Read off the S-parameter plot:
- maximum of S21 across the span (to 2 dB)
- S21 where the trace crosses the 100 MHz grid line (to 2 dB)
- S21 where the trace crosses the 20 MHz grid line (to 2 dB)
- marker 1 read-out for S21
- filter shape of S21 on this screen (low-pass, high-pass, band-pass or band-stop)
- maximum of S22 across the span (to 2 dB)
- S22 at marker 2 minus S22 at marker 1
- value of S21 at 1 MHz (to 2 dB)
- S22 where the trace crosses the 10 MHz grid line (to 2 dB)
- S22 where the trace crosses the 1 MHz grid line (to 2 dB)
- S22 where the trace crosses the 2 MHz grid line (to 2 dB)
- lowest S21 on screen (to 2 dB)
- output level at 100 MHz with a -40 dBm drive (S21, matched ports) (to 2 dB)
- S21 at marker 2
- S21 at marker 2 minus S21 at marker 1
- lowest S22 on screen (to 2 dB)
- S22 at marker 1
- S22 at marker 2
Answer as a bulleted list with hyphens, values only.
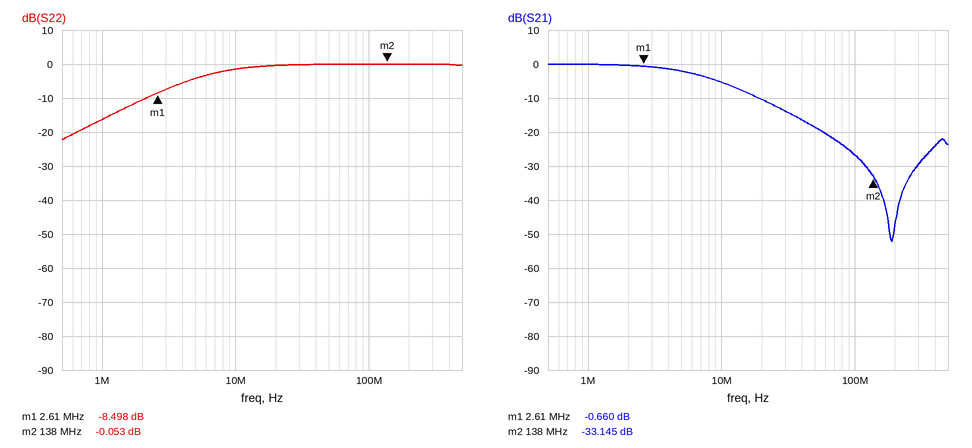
- 0 dB
- -26 dB
- -10 dB
- -0.660 dB
- low-pass
- 0 dB
- 8.445 dB
- 0 dB
- -2 dB
- -16 dB
- -10 dB
- -52 dB
- -66 dBm
- -33.145 dB
- -32.485 dB
- -22 dB
- -8.498 dB
- -0.053 dB
